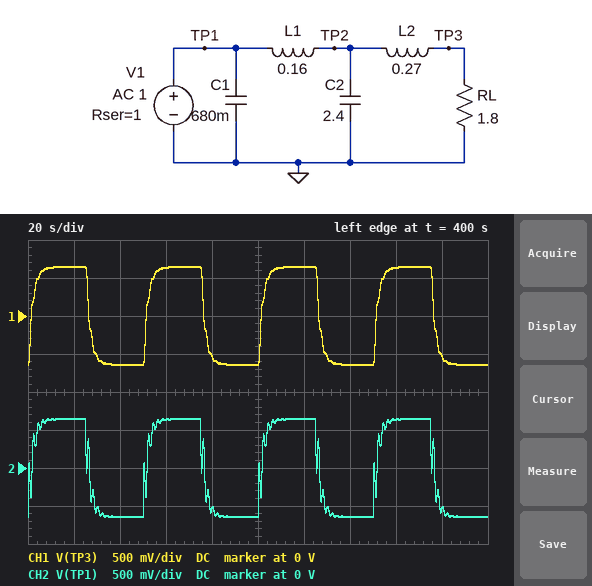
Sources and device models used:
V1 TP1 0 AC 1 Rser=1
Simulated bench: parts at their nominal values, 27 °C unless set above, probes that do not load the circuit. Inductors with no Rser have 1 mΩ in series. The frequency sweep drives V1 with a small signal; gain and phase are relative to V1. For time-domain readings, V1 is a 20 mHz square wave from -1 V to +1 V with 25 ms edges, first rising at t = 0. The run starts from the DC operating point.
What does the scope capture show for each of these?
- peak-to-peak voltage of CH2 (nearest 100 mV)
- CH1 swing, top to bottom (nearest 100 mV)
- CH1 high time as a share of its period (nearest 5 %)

1.3 V
1.3 V
50 %
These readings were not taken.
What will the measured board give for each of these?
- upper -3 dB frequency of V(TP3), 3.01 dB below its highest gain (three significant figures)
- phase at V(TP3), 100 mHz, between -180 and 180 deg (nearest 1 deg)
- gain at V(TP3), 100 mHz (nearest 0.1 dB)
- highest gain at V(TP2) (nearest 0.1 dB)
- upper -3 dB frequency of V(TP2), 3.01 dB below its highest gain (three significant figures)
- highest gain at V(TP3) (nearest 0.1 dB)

88.4 mHz
-59 deg
-7.4 dB
-3.8 dB
89.0 mHz
-3.8 dB
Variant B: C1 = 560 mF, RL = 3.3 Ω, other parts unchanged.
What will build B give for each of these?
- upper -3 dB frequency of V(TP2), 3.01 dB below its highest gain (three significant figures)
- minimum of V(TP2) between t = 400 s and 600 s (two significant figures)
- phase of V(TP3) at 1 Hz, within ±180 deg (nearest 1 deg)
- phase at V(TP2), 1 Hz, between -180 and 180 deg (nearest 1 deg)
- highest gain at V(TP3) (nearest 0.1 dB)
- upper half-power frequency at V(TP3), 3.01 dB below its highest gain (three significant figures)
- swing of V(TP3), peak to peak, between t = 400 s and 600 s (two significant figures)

75.2 mHz
-770 mV
86 deg
113 deg
-2.3 dB
75.1 mHz
1.5 V
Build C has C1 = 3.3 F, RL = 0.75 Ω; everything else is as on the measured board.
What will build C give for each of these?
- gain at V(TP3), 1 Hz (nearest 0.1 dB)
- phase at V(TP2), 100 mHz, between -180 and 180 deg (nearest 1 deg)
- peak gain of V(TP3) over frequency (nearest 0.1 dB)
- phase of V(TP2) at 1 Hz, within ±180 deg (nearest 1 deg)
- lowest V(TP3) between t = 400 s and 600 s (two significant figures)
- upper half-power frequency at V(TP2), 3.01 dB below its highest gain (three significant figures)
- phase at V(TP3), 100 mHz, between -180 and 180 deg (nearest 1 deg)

-56.5 dB
-59 deg
-7.4 dB
94 deg
-440 mV
373 mHz
-72 deg
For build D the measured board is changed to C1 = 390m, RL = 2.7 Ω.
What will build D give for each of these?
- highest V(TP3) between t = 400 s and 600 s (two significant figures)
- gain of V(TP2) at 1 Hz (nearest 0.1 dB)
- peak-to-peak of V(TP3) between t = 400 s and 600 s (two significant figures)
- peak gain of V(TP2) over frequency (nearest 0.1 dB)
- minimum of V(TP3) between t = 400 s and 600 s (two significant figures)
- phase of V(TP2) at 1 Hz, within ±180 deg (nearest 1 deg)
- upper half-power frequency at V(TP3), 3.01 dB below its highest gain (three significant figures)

730 mV
-27.6 dB
1.5 V
-2.7 dB
-730 mV
127 deg
84.5 mHz
